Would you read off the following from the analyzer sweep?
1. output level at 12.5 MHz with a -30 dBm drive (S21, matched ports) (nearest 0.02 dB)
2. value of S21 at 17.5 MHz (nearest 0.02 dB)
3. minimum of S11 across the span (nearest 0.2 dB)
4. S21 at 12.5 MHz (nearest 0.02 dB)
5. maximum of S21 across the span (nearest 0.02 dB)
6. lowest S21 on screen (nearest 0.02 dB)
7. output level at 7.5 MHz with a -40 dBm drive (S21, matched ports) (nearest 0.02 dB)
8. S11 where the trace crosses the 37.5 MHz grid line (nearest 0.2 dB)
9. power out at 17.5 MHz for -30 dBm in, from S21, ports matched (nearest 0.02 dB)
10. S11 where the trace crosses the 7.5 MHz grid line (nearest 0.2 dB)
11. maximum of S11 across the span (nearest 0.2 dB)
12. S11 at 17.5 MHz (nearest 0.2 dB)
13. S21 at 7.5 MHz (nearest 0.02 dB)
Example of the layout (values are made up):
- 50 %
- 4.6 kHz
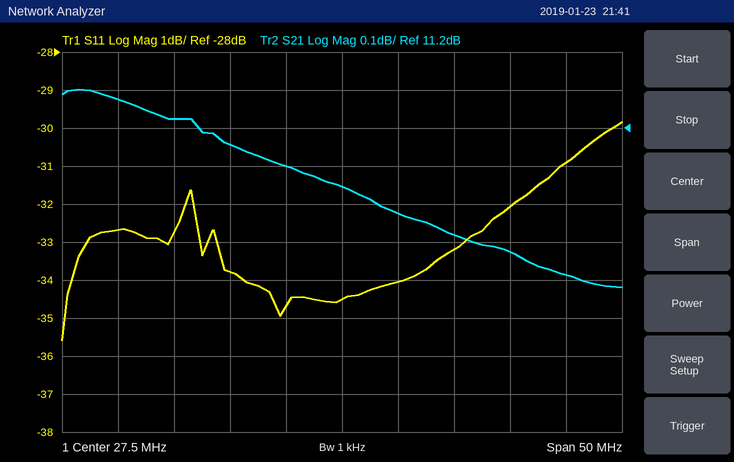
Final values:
- -18.78 dBm
- 11.16 dB
- -35.6 dB
- 11.22 dB
- 11.30 dB
- 10.78 dB
- -28.72 dBm
- -33.2 dB
- -18.84 dBm
- -32.6 dB
- -29.8 dB
- -33.8 dB
- 11.28 dB
